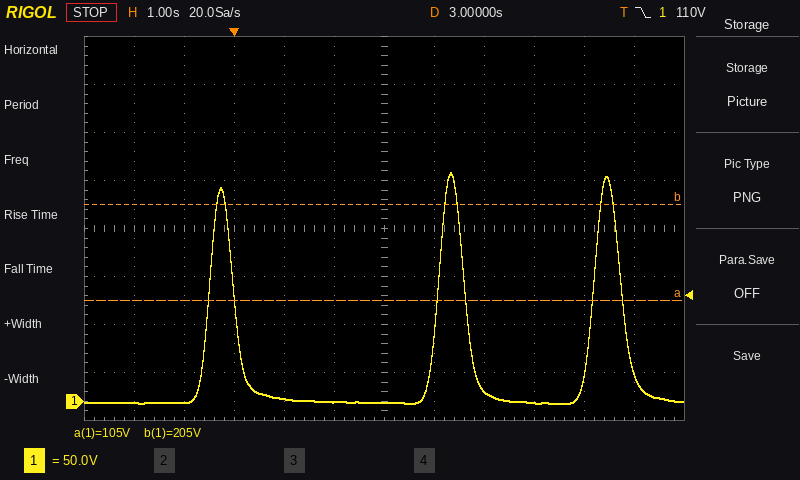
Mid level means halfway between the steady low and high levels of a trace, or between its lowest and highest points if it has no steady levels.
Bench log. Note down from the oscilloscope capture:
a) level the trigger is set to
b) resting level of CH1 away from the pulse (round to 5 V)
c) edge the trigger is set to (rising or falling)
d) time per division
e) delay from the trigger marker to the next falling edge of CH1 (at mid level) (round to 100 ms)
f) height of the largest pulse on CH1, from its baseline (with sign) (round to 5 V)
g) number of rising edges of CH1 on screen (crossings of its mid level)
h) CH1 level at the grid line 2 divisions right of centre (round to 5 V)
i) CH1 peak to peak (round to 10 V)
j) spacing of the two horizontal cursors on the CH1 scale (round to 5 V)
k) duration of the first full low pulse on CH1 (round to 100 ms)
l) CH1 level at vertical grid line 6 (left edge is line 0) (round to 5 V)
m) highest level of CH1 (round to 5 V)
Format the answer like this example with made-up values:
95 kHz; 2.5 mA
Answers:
110 V; 0 V; falling; 1 s; 4.6 s; +240 V; 3; 10 V; 240 V; 100 V; 4.1 s; 0 V; 240 V
